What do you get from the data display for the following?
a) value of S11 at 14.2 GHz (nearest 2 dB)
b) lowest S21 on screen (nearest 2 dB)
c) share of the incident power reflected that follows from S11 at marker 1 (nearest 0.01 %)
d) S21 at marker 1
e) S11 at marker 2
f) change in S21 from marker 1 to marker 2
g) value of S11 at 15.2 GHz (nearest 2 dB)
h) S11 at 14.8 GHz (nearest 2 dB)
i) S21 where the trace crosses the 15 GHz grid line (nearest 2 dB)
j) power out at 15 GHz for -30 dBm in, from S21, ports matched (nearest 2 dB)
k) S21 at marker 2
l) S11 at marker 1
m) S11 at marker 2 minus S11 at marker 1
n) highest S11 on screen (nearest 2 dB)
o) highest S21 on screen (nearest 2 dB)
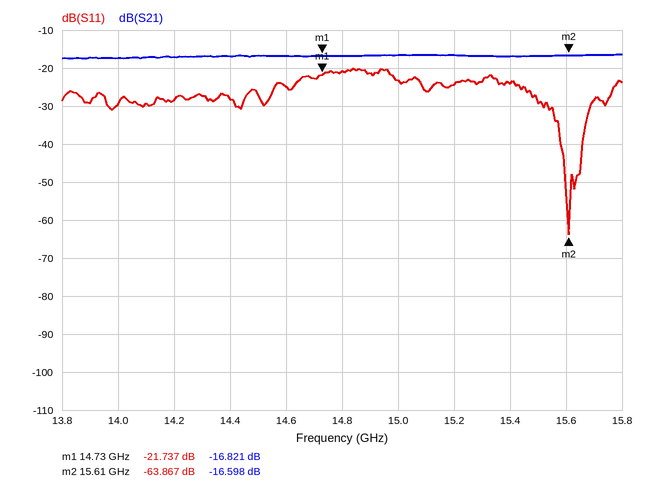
-28 dB
-18 dB
0.67 %
-16.821 dB
-63.867 dB
0.223 dB
-24 dB
-20 dB
-16 dB
-46 dBm
-16.598 dB
-21.737 dB
-42.130 dB
-20 dB
-16 dB
